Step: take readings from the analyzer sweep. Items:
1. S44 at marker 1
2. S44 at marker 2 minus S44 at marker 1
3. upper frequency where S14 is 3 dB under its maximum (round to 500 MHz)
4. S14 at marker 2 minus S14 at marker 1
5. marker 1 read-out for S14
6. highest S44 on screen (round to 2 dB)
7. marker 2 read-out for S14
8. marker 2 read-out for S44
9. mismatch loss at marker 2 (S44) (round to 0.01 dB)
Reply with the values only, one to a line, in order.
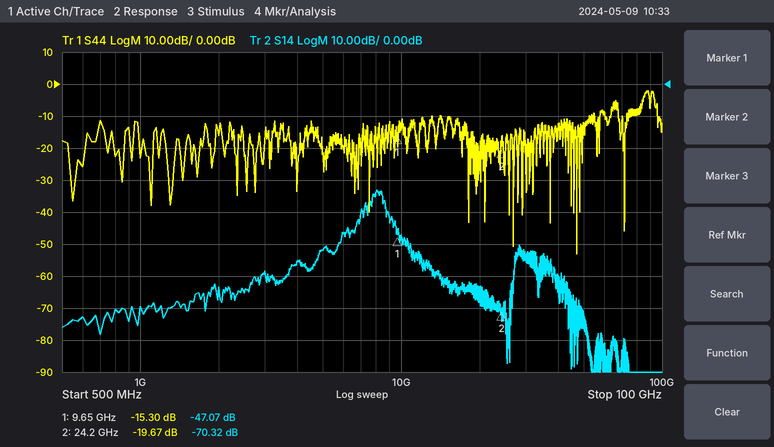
-15.30 dB
-4.37 dB
8.5 GHz
-23.25 dB
-47.07 dB
-2 dB
-70.32 dB
-19.67 dB
0.05 dB
